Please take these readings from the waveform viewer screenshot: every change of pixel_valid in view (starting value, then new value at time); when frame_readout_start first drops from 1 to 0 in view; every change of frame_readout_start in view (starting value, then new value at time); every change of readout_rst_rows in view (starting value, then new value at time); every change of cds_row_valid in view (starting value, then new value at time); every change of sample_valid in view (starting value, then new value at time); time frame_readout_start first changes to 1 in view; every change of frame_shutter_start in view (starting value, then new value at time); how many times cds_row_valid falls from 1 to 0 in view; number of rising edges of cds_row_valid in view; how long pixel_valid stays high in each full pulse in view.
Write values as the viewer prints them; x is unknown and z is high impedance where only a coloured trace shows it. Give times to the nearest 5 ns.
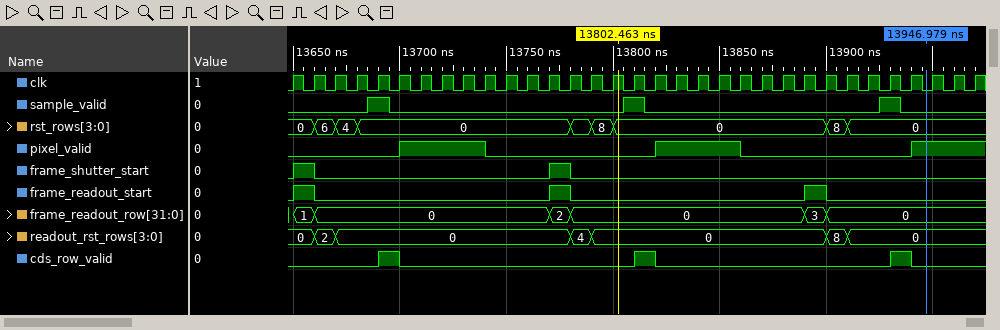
0, 1 at 13700 ns, 0 at 13740 ns, 1 at 13820 ns, 0 at 13860 ns, 1 at 13940 ns
13660 ns
0, 1 at 13650 ns, 0 at 13660 ns, 1 at 13770 ns, 0 at 13780 ns, 1 at 13890 ns, 0 at 13900 ns
0, 2 at 13660 ns, 0 at 13670 ns, 4 at 13780 ns, 0 at 13790 ns, 8 at 13900 ns, 0 at 13910 ns
0, 1 at 13690 ns, 0 at 13700 ns, 1 at 13810 ns, 0 at 13820 ns, 1 at 13930 ns, 0 at 13940 ns
0, 1 at 13685 ns, 0 at 13695 ns, 1 at 13805 ns, 0 at 13815 ns, 1 at 13925 ns, 0 at 13935 ns
13650 ns
0, 1 at 13650 ns, 0 at 13660 ns, 1 at 13770 ns, 0 at 13780 ns
3
3
40 ns, 40 ns
